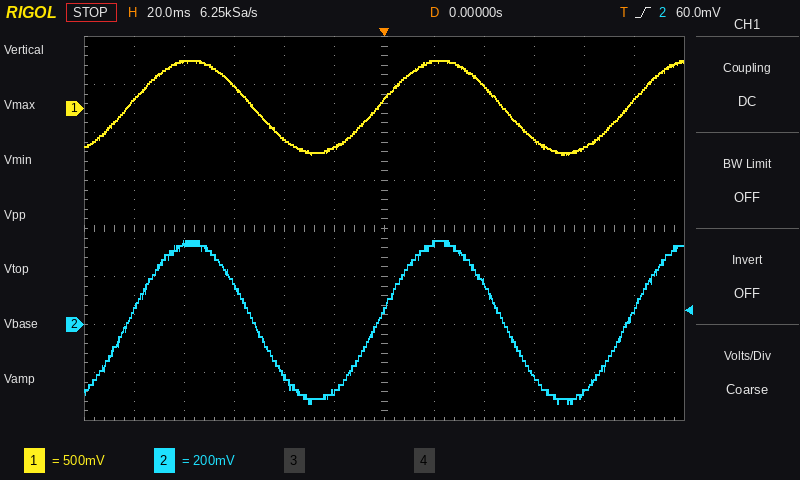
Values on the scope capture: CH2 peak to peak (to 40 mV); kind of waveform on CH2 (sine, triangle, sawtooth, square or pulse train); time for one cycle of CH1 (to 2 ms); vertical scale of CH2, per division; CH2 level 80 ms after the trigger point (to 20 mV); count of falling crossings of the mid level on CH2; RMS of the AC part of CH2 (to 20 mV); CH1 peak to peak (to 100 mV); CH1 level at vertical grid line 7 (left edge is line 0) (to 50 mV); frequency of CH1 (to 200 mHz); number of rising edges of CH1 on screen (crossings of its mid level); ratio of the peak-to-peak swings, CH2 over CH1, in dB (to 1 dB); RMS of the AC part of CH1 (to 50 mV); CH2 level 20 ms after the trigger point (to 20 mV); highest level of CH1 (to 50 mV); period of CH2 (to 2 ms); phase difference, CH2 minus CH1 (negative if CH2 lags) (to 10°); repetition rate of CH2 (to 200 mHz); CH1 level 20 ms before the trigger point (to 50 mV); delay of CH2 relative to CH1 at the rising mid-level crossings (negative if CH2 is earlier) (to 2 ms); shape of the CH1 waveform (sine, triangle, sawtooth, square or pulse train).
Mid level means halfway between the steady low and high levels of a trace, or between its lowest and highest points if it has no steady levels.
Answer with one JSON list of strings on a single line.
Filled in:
["680 mV", "sine", "100 ms", "200 mV", "-280 mV", "2", "240 mV", "1.00 V", "500 mV", "10.0 Hz", "3", "-3 dB", "350 mV", "340 mV", "500 mV", "100 ms", "0°", "10.0 Hz", "-400 mV", "0 ms", "sine"]
